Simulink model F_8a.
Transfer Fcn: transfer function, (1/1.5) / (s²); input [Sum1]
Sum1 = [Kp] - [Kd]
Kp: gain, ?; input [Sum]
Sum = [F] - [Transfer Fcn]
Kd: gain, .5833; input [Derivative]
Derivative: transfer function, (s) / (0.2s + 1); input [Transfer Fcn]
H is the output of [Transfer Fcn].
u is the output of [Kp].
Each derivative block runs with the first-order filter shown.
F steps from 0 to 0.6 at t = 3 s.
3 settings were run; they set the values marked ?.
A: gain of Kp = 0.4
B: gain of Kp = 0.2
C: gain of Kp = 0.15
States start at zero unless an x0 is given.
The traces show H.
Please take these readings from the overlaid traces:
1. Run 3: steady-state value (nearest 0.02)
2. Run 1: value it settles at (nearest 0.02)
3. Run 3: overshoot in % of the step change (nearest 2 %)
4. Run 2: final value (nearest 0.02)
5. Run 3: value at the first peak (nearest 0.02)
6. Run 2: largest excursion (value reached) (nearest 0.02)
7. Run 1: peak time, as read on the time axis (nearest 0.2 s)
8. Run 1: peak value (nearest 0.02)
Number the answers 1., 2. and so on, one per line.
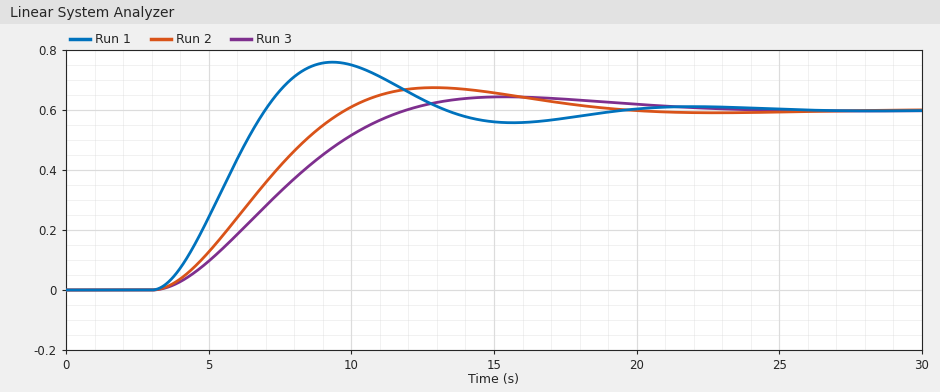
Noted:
1. 0.60
2. 0.60
3. 8 %
4. 0.60
5. 0.64
6. 0.68
7. 9.4 s
8. 0.76
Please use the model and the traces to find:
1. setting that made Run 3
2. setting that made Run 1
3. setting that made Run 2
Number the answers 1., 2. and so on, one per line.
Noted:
1. C
2. A
3. B
